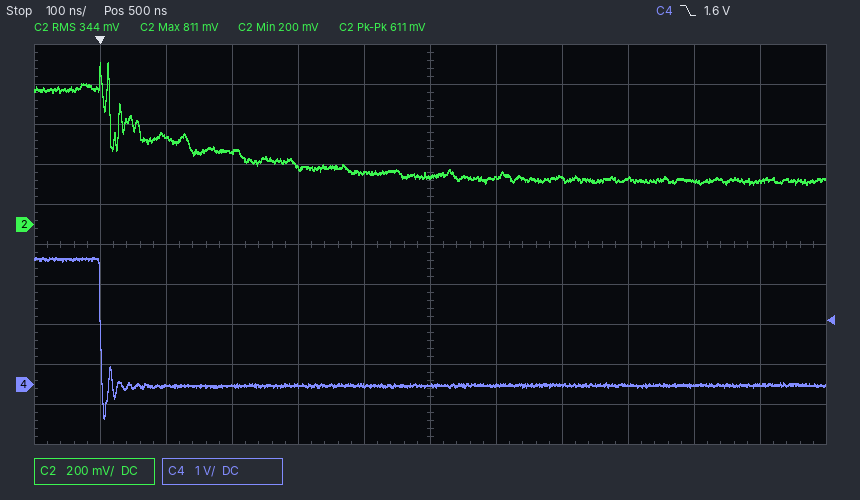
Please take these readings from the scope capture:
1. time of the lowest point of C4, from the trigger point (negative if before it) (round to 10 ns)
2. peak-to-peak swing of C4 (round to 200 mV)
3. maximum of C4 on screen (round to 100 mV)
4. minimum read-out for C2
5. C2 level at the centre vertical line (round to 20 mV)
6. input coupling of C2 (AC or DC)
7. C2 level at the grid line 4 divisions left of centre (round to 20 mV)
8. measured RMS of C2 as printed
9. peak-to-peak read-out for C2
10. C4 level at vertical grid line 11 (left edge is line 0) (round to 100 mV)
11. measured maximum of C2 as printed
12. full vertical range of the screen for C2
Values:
+10 ns
4.0 V
3.2 V
200 mV
240 mV
DC
440 mV
344 mV
611 mV
0.0 V
811 mV
2 V
